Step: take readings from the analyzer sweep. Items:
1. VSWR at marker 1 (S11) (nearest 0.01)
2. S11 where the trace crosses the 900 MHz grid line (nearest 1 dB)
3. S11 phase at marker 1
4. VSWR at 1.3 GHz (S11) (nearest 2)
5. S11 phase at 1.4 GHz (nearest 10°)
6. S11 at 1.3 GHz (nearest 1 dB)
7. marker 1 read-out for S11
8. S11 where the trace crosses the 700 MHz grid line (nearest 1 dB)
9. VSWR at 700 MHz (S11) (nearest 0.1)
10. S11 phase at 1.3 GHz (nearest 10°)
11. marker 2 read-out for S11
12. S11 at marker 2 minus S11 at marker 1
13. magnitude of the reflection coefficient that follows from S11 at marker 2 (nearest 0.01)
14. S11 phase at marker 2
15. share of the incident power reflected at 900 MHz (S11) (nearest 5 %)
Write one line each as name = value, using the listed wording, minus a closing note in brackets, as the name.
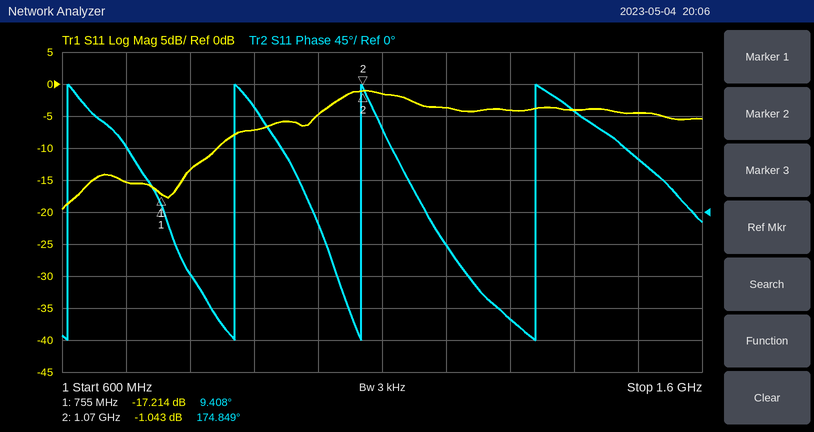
VSWR at marker 1 (S11) = 1.32
S11 where the trace crosses the 900 MHz grid line = -7 dB
S11 phase at marker 1 = 9.408°
VSWR at 1.3 GHz (S11) = 4
S11 phase at 1.4 GHz = 140°
S11 at 1.3 GHz = -4 dB
marker 1 read-out for S11 = -17.214 dB
S11 where the trace crosses the 700 MHz grid line = -15 dB
VSWR at 700 MHz (S11) = 1.4
S11 phase at 1.3 GHz = -150°
marker 2 read-out for S11 = -1.043 dB
S11 at marker 2 minus S11 at marker 1 = 16.171 dB
magnitude of the reflection coefficient that follows from S11 at marker 2 = 0.89
S11 phase at marker 2 = 174.849°
share of the incident power reflected at 900 MHz (S11) = 20 %
